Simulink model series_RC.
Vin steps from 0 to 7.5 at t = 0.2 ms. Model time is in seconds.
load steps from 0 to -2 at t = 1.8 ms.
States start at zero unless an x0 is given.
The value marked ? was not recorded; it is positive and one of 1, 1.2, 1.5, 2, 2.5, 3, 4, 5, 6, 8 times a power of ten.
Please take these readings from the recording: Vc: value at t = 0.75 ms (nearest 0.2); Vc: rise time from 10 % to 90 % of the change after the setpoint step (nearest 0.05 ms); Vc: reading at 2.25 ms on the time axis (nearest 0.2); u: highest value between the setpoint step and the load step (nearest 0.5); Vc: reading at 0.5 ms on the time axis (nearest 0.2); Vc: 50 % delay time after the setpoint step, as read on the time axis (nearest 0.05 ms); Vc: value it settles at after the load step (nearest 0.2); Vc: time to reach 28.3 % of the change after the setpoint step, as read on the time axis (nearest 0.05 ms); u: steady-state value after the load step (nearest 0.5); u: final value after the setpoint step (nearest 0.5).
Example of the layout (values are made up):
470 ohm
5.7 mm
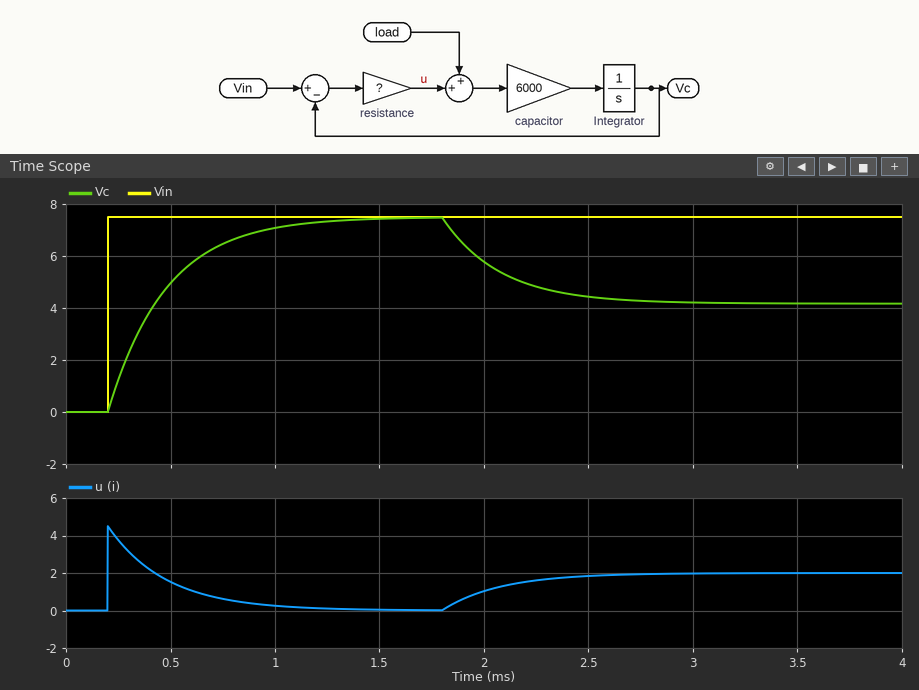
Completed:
6.4
0.60 ms
4.8
4.5
5.0
0.40 ms
4.2
0.30 ms
2.0
0.0
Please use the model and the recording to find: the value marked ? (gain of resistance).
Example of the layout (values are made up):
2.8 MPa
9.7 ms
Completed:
0.6
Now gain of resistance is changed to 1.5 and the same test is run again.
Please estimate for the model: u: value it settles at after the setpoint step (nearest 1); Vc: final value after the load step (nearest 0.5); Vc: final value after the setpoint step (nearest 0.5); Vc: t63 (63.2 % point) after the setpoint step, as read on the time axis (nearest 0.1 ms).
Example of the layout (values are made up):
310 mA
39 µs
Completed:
0
6.0
7.5
0.3 ms
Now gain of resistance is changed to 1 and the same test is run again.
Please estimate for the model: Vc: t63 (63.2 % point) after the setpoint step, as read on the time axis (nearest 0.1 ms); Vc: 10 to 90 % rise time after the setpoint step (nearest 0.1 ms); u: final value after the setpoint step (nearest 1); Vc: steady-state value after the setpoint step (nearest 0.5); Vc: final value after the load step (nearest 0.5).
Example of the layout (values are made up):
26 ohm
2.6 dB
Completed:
0.4 ms
0.4 ms
0
7.5
5.5
